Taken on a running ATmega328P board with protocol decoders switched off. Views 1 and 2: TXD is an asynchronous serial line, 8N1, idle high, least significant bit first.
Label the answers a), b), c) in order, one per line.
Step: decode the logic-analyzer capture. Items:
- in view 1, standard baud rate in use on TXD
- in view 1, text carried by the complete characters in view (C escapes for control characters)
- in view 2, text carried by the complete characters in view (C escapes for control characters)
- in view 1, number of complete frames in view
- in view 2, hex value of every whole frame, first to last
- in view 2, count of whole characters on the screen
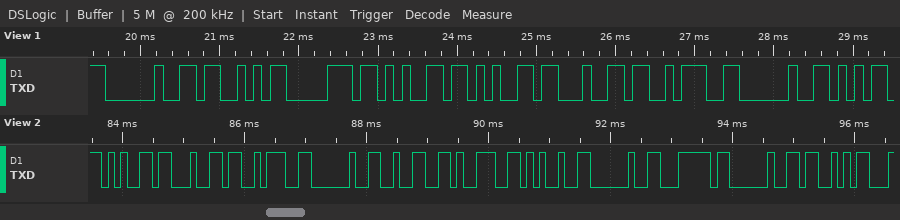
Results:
a) 9600 baud
b) " Speed: "
c) "ed: 29% | S"
d) 8
e) 0x65 0x64 0x3A 0x20 0x32 0x39 0x25 0x20 0x7C 0x20 0x53
f) 11
